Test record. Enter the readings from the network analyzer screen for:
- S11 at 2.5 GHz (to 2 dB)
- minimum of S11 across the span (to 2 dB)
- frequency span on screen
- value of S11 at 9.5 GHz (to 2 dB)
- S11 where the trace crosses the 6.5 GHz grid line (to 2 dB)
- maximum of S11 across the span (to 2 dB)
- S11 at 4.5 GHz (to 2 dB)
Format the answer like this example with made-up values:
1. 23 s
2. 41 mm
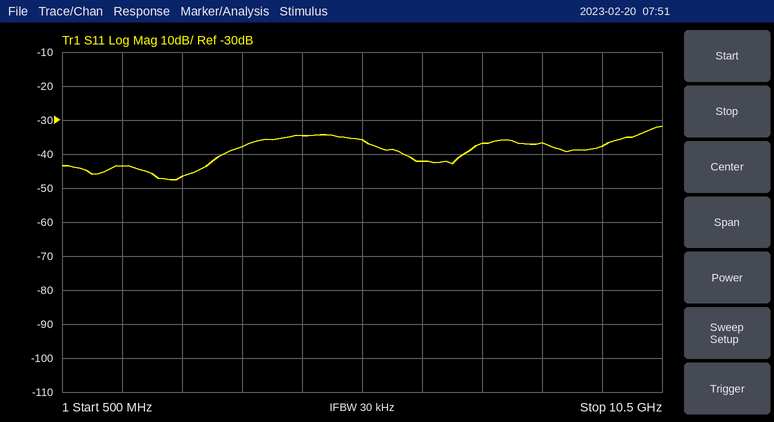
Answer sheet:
1. -46 dB
2. -48 dB
3. 10 GHz
4. -38 dB
5. -42 dB
6. -32 dB
7. -34 dB
